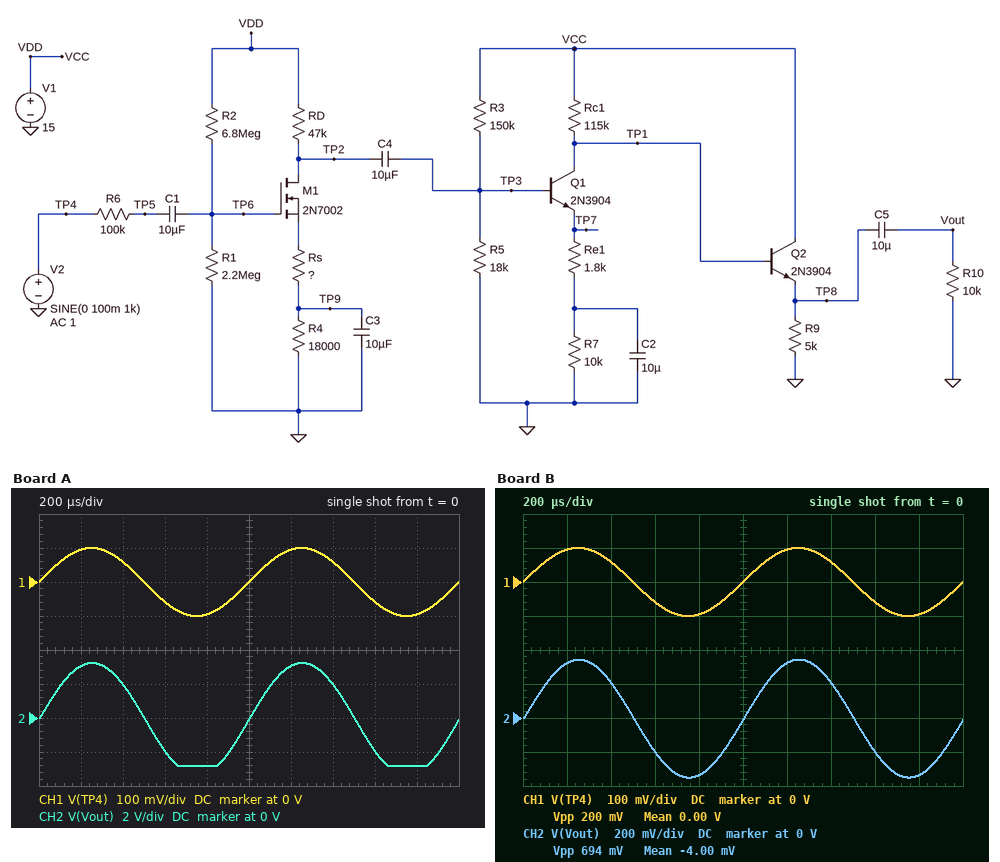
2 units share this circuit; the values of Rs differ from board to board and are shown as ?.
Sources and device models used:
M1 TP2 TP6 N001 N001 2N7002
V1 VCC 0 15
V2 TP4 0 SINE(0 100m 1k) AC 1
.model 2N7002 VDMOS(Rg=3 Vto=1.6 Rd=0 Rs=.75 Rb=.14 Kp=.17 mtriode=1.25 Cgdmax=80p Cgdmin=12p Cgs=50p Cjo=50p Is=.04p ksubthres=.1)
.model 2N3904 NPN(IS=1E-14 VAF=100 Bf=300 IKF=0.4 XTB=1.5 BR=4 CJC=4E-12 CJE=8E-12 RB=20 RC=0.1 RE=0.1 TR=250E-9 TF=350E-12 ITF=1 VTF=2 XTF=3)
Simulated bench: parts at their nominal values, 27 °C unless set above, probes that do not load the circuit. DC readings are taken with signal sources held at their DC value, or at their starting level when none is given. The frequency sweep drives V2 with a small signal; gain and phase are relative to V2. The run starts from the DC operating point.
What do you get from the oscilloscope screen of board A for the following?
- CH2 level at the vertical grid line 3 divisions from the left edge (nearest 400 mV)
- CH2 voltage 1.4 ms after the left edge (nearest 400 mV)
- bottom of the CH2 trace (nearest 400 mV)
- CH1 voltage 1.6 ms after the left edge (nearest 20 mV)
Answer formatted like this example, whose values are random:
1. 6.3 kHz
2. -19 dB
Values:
1. -2.0 V
2. 2.0 V
3. -2.8 V
4. -60 mV
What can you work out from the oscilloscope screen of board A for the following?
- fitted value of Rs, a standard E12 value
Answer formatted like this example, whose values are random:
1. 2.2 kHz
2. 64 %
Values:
1. 15 kΩ
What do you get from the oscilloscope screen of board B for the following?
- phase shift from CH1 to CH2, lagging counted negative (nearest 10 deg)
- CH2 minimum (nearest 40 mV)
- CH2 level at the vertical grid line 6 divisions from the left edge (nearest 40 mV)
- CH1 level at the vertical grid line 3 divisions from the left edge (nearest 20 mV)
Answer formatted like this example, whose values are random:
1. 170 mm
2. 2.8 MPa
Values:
1. 0 deg
2. -360 mV
3. 320 mV
4. -60 mV
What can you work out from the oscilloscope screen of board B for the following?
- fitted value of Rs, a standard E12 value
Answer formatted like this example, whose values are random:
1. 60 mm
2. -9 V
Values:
1. 150 kΩ
